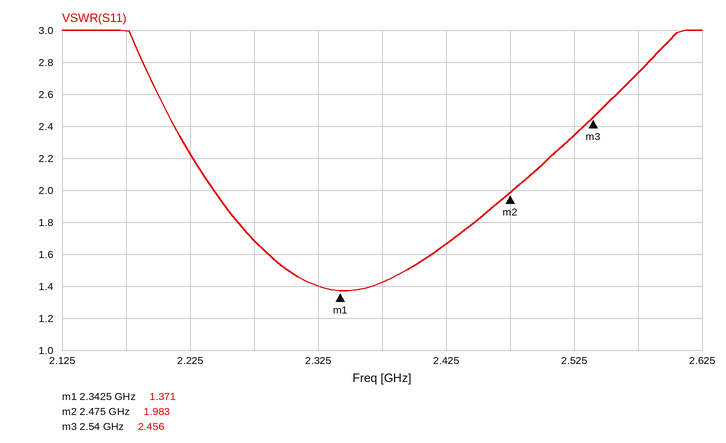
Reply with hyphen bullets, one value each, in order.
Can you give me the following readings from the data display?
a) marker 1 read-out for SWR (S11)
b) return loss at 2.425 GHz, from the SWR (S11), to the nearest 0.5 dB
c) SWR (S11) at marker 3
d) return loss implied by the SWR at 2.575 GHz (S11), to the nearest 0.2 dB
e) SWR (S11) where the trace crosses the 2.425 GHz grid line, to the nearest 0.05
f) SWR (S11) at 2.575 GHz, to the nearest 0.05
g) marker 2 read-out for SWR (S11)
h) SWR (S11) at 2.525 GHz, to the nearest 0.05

- 1.371
- 12.0 dB
- 2.456
- 6.6 dB
- 1.65
- 2.75
- 1.983
- 2.35
